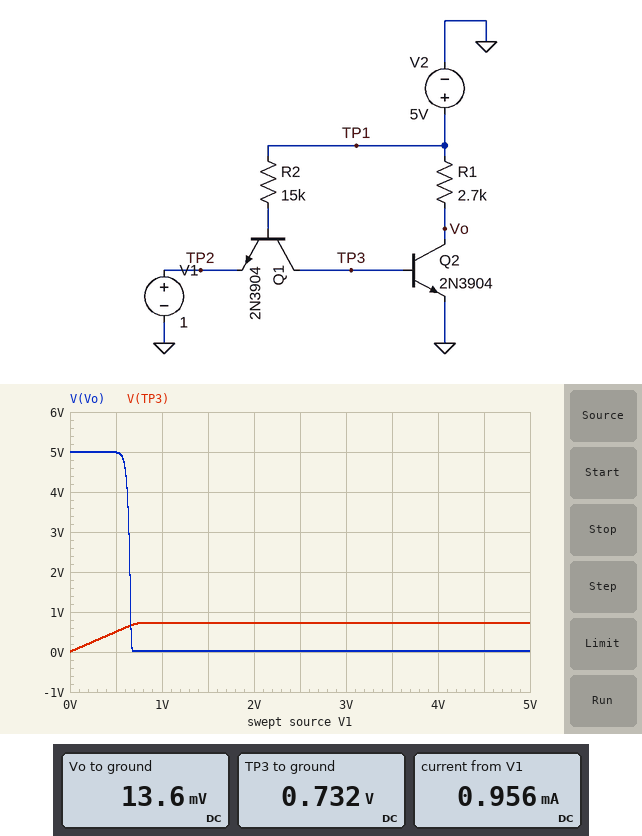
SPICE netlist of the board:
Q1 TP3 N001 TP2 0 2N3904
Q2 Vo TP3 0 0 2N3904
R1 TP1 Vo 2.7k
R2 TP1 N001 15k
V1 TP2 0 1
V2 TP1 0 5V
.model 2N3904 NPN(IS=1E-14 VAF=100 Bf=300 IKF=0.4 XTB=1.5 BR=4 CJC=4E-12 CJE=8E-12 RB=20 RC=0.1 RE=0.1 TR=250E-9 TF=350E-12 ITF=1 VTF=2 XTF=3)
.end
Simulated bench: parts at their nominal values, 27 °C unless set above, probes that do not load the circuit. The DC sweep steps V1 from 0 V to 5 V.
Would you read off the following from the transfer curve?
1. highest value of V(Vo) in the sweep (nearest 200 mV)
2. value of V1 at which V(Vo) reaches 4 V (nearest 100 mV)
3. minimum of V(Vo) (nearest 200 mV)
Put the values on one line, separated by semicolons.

5.0 V; 600 mV; 0 V
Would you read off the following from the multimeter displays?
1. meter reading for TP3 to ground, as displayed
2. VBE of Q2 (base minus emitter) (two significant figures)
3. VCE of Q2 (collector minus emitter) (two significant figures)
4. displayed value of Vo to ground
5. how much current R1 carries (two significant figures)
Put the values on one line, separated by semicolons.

0.732 V; 730 mV; 14 mV; 13.6 mV; 1.8 mA
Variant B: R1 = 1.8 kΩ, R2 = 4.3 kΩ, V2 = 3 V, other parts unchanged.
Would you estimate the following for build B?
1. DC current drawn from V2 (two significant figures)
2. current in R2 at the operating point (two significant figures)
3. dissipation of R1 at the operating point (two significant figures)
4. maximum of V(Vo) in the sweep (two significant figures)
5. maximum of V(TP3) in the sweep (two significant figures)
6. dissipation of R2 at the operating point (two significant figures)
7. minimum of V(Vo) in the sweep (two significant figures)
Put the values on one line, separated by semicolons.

2.0 mA; 370 µA; 5.0 mW; 3.0 V; 750 mV; 580 µW; 11 mV
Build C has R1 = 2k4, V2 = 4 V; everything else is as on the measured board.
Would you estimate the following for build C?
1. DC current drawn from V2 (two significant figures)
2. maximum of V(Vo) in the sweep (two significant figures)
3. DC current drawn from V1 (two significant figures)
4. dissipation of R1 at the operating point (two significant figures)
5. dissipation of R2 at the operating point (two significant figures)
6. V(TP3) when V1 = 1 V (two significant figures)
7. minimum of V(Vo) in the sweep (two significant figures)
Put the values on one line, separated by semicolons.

1.8 mA; 4.0 V; 700 µA; 6.6 mW; 460 µW; 720 mV; 15 mV
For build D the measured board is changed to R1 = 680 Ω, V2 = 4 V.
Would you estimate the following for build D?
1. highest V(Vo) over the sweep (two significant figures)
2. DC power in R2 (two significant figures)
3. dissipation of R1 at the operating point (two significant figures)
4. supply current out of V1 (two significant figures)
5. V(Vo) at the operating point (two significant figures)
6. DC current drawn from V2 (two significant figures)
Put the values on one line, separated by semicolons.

4.0 V; 460 µW; 23 mW; 690 µA; 30 mV; 6.0 mA
